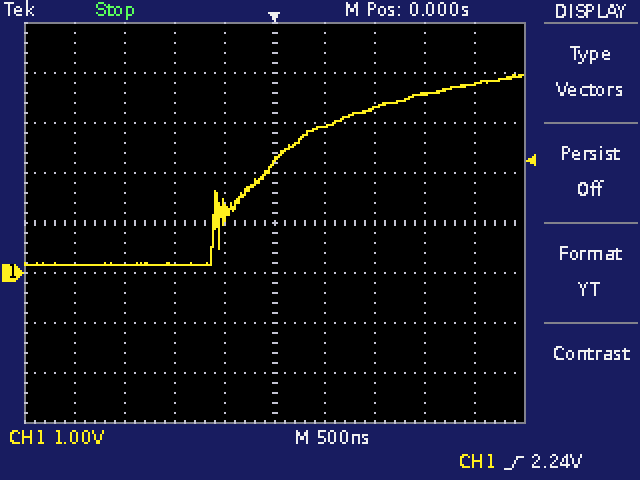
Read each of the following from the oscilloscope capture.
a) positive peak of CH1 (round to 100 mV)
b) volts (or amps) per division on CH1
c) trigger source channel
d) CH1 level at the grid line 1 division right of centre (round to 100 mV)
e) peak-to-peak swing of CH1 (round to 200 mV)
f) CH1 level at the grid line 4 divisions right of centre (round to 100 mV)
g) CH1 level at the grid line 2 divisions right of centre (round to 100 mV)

4.0 V
1 V
CH1
2.9 V
3.8 V
3.8 V
3.3 V
